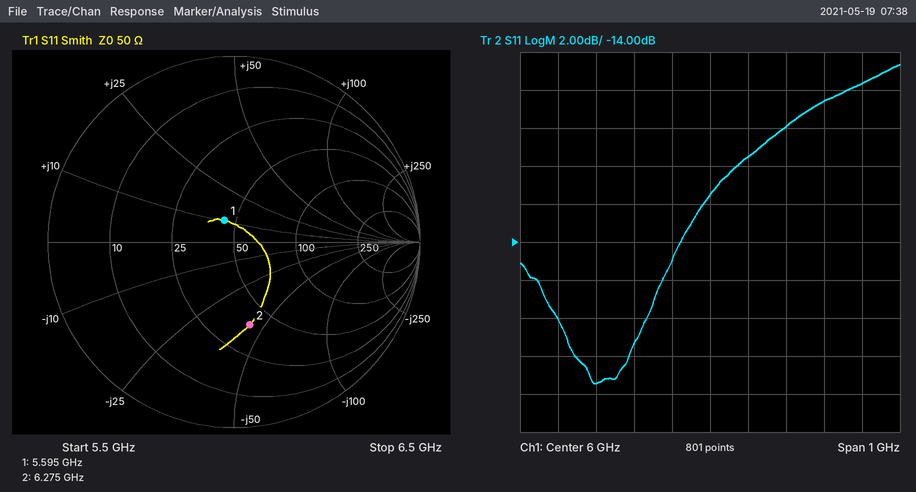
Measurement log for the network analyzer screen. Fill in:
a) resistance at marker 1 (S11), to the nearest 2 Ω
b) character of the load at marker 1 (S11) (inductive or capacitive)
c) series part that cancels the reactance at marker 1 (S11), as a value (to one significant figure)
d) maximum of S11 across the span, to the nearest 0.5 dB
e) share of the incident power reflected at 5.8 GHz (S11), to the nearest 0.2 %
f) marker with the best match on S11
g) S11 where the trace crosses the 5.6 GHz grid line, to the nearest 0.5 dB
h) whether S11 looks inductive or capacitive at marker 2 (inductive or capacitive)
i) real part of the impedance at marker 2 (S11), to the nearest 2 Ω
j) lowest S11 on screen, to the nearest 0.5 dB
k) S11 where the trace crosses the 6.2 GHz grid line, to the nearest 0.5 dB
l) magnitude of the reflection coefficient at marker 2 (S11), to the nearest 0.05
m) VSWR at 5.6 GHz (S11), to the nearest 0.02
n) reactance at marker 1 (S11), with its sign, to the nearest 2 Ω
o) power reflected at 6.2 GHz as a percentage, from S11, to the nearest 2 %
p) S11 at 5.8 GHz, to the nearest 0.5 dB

44 Ω
inductive
3 pF
-4.5 dB
1.2 %
marker 1
-18.0 dB
capacitive
38 Ω
-21.5 dB
-8.0 dB
0.45
1.28
+10 Ω
16 %
-19.5 dB
